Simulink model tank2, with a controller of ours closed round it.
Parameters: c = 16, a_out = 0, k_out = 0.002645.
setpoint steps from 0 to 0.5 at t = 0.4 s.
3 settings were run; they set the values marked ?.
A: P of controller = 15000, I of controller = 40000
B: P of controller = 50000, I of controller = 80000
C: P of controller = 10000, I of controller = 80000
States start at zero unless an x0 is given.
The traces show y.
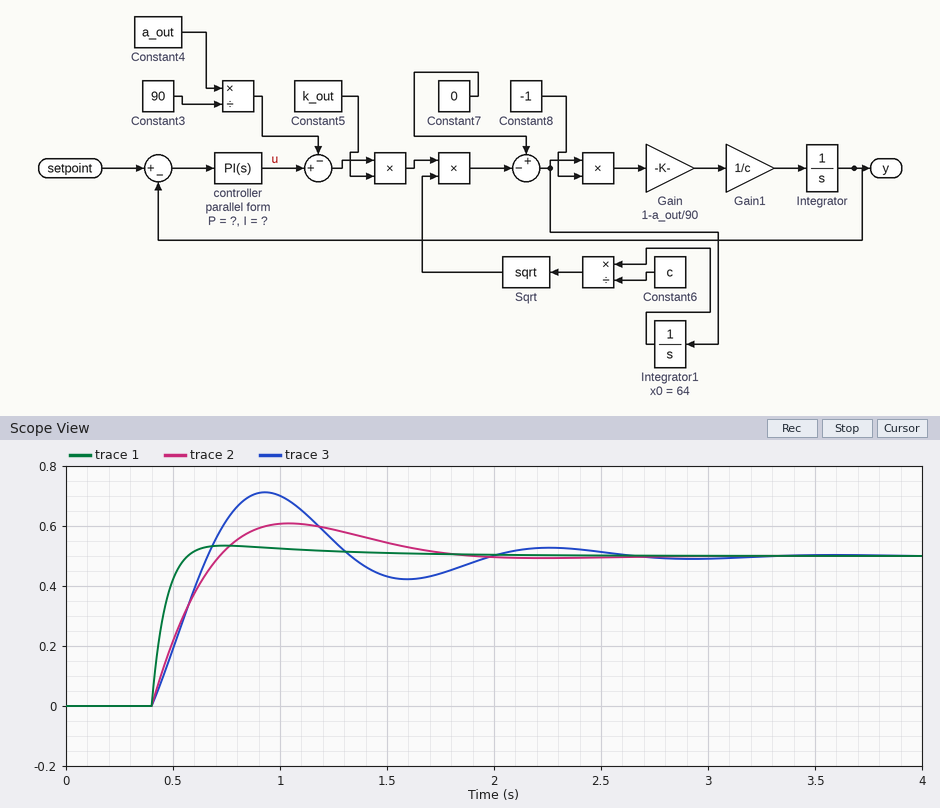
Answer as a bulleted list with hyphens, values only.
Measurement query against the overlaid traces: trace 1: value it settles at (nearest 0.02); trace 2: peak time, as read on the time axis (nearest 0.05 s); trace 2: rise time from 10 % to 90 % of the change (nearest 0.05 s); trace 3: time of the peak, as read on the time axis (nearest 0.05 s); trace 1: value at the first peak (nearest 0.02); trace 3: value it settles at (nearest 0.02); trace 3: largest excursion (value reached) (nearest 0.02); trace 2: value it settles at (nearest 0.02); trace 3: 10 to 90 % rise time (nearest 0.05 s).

- 0.50
- 1.05 s
- 0.25 s
- 0.95 s
- 0.54
- 0.50
- 0.72
- 0.50
- 0.20 s
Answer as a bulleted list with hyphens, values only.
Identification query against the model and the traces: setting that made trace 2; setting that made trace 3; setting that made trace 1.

- A
- C
- B
